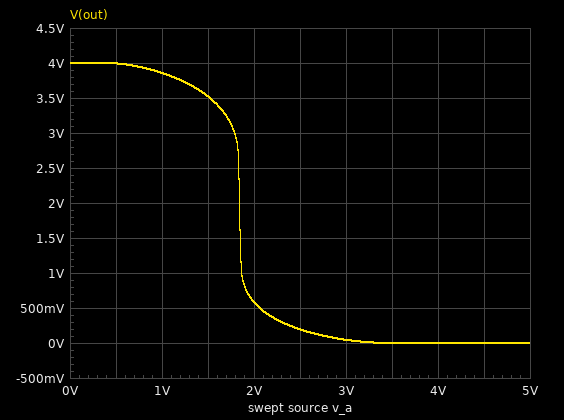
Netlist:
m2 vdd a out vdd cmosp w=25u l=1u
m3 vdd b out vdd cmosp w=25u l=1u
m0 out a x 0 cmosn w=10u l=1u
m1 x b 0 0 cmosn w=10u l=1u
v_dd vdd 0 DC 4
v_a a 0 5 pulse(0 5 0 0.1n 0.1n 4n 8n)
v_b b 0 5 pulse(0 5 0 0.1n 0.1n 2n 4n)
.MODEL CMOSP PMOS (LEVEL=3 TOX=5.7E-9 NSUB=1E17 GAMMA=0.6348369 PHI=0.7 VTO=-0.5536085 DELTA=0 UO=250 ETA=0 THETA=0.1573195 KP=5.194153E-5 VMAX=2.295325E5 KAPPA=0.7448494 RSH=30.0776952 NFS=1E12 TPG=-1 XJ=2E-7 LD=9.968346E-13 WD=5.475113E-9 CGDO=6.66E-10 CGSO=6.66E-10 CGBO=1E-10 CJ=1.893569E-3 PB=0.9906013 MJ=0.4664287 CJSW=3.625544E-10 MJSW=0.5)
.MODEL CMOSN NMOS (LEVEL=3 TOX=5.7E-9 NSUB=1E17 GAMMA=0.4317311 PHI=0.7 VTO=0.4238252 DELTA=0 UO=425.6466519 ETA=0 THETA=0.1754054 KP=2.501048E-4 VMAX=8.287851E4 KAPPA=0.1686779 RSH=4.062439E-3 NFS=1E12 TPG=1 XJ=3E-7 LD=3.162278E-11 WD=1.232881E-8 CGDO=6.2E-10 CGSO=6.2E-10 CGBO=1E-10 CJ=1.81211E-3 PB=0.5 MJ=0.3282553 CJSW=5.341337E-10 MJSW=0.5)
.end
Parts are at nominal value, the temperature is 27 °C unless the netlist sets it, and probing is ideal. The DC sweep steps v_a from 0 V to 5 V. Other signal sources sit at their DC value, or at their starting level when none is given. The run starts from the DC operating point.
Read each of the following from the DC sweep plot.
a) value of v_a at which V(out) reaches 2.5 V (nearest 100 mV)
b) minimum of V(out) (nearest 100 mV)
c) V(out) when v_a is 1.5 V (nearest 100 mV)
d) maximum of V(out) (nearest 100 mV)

1.8 V
0 V
3.5 V
4.0 V
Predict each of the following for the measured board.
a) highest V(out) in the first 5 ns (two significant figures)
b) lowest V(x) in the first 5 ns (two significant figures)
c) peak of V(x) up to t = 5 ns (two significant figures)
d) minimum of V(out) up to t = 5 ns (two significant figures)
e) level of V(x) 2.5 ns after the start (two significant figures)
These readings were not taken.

4.7 V
-630 mV
4.1 V
-610 mV
3.7 V
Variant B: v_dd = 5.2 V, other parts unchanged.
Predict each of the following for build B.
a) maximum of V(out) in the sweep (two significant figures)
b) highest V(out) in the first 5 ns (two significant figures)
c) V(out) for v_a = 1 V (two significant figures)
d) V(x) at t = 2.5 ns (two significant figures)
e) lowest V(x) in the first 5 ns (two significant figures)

5.2 V
5.9 V
5.1 V
4.0 V
-420 mV
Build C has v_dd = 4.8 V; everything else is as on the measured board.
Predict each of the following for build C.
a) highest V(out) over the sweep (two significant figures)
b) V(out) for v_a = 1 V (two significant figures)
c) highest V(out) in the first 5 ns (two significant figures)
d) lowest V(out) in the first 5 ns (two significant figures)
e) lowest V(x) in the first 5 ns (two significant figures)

4.8 V
4.7 V
5.5 V
-430 mV
-500 mV
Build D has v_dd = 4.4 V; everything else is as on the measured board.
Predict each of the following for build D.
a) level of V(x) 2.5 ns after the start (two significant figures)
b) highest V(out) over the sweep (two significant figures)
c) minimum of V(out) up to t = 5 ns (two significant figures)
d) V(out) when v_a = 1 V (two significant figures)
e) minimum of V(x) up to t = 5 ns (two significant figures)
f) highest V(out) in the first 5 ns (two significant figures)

3.9 V
4.4 V
-490 mV
4.3 V
-600 mV
5.1 V
